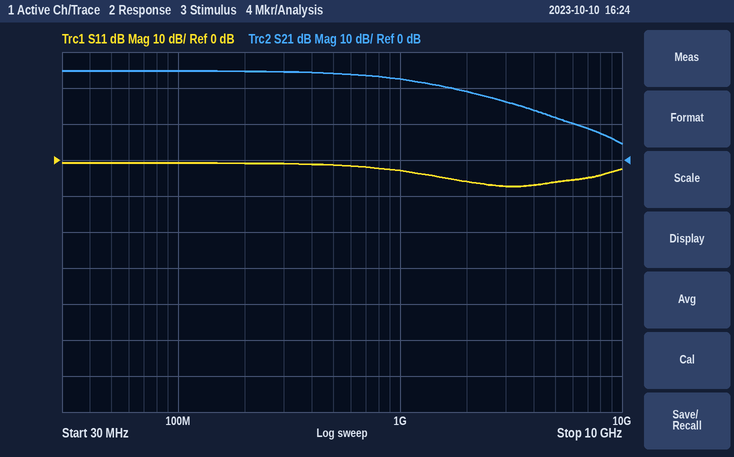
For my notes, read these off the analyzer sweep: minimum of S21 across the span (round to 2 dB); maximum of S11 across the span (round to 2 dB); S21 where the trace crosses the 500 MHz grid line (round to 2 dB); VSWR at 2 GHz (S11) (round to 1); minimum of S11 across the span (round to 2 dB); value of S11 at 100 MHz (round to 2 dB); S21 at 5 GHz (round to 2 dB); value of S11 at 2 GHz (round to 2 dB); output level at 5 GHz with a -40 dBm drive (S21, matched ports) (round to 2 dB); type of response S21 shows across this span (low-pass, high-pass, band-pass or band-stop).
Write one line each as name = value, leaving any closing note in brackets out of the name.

minimum of S21 across the span = 4 dB
maximum of S11 across the span = 0 dB
S21 where the trace crosses the 500 MHz grid line = 24 dB
VSWR at 2 GHz (S11) = 3
minimum of S11 across the span = -8 dB
value of S11 at 100 MHz = 0 dB
S21 at 5 GHz = 12 dB
value of S11 at 2 GHz = -6 dB
output level at 5 GHz with a -40 dBm drive (S21, matched ports) = -28 dBm
type of response S21 shows across this span = low-pass
